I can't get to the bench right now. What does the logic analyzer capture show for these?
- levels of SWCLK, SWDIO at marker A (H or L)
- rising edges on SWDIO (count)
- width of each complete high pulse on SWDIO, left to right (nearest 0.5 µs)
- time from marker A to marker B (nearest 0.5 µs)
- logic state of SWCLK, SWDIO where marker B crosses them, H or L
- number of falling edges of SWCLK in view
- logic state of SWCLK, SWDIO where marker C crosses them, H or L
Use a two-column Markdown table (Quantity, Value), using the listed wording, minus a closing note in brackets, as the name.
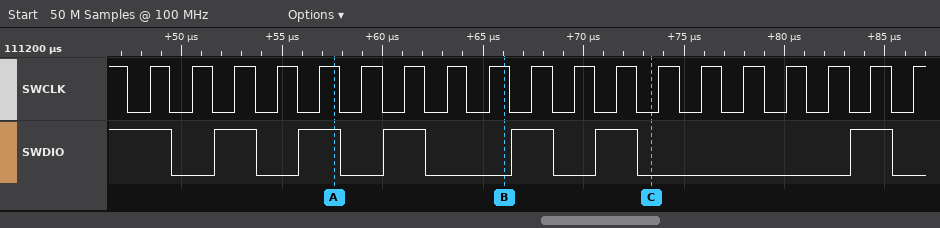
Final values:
| Quantity | Value |
|---|---|
| levels of SWCLK, SWDIO at marker A | SWCLK=H, SWDIO=H |
| rising edges on SWDIO | 6 |
| width of each complete high pulse on SWDIO, left to right | 2 µs, 2 µs, 2 µs, 2 µs, 2 µs, 2 µs |
| time from marker A to marker B | 8.5 µs |
| logic state of SWCLK, SWDIO where marker B crosses them, H or L | SWCLK=H, SWDIO=L |
| number of falling edges of SWCLK in view | 19 |
| logic state of SWCLK, SWDIO where marker C crosses them, H or L | SWCLK=L, SWDIO=L |
